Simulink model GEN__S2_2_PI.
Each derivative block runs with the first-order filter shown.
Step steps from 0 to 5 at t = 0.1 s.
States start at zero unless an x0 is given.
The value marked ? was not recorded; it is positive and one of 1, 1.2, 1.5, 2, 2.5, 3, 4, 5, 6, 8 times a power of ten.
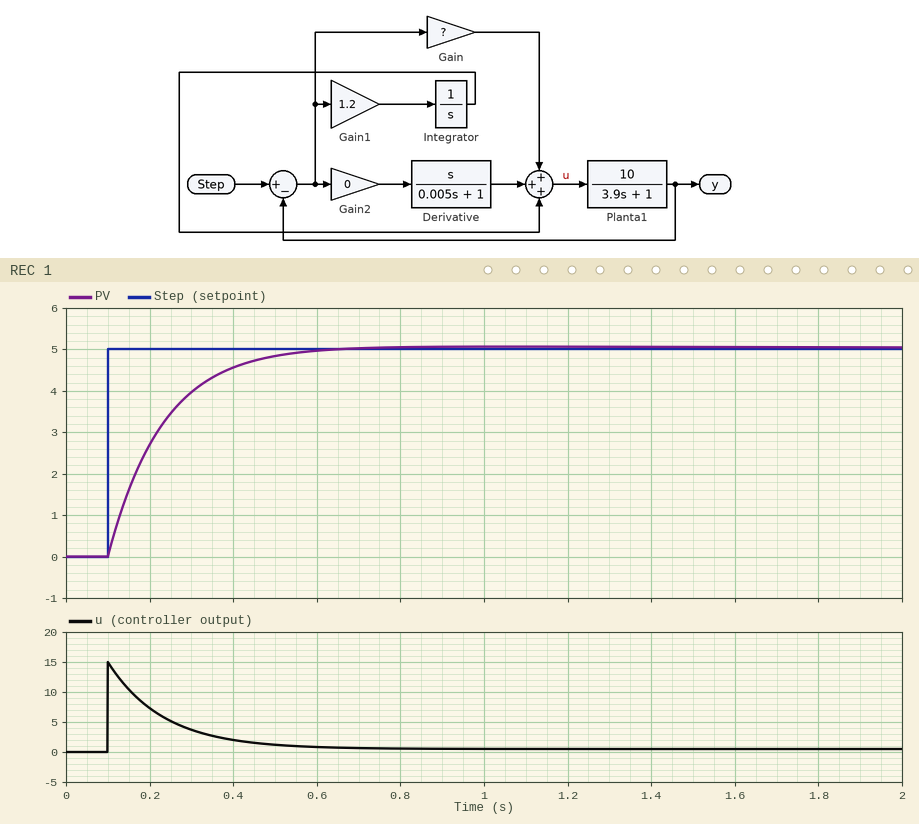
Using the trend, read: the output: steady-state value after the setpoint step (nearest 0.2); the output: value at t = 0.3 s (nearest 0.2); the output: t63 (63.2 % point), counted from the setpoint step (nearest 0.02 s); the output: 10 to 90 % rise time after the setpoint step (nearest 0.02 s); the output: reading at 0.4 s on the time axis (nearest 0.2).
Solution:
5.0
4.0
0.12 s
0.28 s
4.6
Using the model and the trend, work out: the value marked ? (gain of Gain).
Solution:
3
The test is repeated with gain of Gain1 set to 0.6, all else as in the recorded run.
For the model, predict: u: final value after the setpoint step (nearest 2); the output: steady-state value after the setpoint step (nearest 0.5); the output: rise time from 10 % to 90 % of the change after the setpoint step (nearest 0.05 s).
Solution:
0
5.0
0.30 s
